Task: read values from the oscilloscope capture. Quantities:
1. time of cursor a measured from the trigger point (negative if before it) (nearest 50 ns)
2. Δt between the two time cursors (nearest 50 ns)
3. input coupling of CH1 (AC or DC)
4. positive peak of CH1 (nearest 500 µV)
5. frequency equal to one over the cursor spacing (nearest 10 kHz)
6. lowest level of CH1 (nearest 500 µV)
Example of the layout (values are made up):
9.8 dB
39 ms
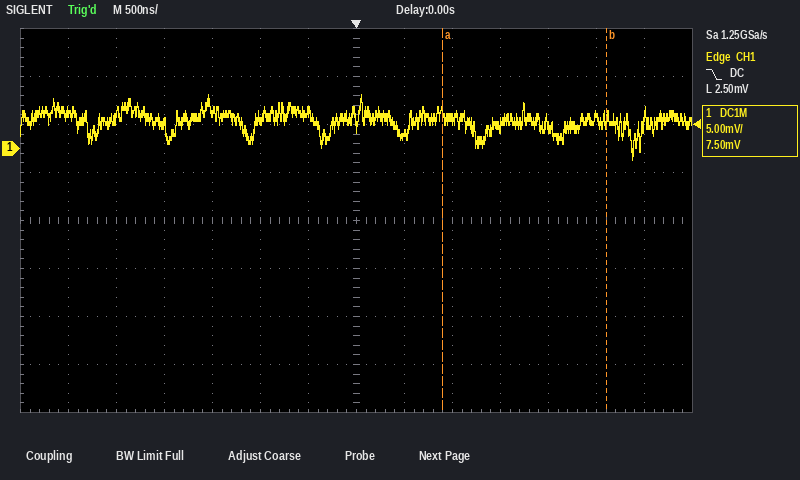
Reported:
+900 ns
1.70 µs
DC
5.5 mV
590 kHz
-1.0 mV
